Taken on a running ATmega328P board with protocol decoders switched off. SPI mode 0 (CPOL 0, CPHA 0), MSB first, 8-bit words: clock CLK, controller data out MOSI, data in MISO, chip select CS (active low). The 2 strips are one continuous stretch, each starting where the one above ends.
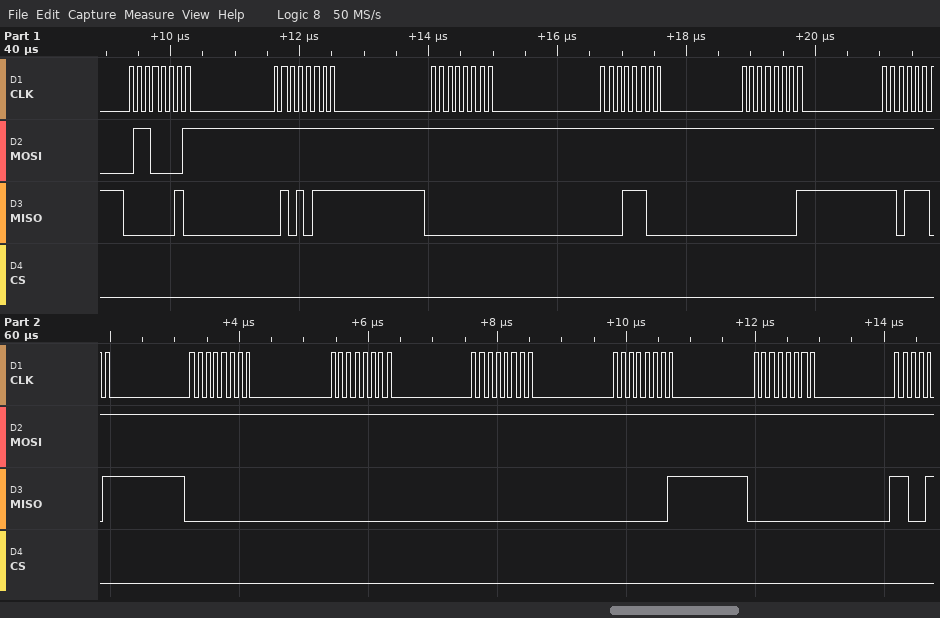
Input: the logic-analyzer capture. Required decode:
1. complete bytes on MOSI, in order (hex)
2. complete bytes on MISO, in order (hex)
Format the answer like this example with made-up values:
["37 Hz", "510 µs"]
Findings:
["0x61 0xFF 0xFF 0xFF 0xFF 0xFF 0xFF 0xFF 0xFF 0xFF 0xFF", "0x02 0x57 0x00 0x1C 0x01 0xDD 0x00 0x00 0x00 0x01 0x00"]
